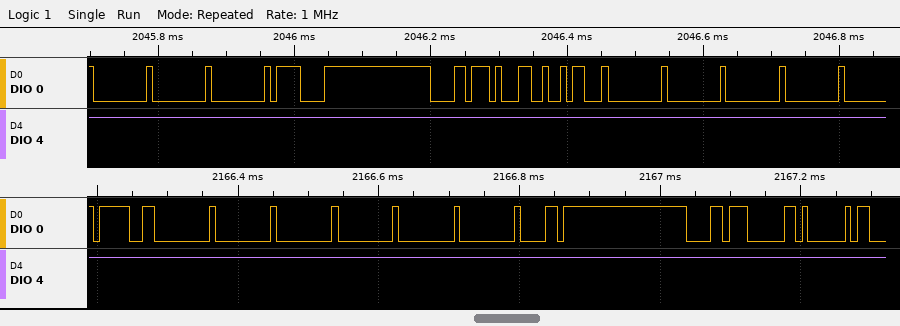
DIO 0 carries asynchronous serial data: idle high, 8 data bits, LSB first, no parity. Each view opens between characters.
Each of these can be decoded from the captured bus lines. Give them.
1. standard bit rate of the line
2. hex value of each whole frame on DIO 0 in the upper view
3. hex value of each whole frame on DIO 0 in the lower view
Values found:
115200 baud
00, 00, 00, 0F, D8, 31, 1A, 00, 00, 00, 00
9F, 00, 00, 00, 00, 00, 00, D8, D8, 60, A0
